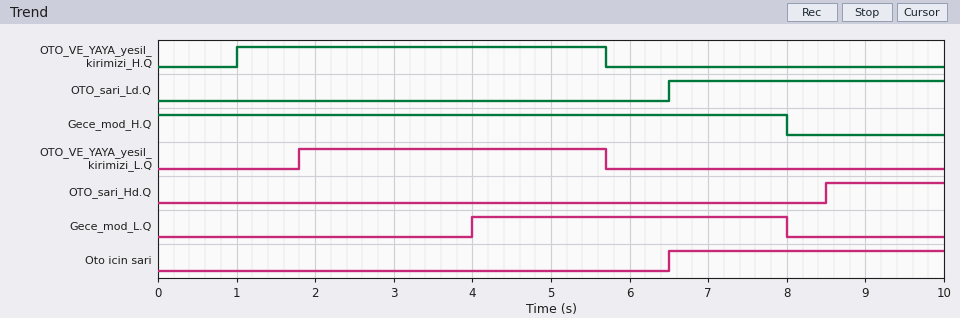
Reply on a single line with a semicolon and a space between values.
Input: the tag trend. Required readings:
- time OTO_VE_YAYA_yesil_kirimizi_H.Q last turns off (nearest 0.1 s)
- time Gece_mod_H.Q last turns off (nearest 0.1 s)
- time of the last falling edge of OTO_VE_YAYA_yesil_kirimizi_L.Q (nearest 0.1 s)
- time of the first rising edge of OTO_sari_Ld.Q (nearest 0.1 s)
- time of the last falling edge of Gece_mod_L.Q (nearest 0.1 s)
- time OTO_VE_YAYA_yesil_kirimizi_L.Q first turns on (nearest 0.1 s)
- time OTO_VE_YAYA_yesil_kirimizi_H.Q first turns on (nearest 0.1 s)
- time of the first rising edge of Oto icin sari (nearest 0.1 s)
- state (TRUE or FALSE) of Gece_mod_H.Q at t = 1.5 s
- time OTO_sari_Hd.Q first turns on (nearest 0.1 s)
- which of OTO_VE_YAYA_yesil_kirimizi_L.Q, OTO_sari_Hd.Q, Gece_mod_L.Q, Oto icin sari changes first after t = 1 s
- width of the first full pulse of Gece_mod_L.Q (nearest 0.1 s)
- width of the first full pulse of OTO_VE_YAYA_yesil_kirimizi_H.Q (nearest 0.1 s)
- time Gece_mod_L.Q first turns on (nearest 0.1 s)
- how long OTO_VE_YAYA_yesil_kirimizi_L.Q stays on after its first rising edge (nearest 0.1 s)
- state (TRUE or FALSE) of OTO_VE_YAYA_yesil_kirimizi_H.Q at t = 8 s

5.7 s; 8.0 s; 5.7 s; 6.5 s; 8.0 s; 1.8 s; 1.0 s; 6.5 s; TRUE; 8.5 s; OTO_VE_YAYA_yesil_kirimizi_L.Q; 4.0 s; 4.7 s; 4.0 s; 3.9 s; FALSE
